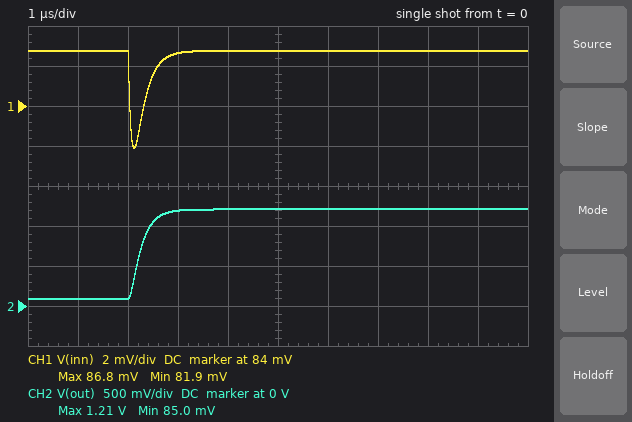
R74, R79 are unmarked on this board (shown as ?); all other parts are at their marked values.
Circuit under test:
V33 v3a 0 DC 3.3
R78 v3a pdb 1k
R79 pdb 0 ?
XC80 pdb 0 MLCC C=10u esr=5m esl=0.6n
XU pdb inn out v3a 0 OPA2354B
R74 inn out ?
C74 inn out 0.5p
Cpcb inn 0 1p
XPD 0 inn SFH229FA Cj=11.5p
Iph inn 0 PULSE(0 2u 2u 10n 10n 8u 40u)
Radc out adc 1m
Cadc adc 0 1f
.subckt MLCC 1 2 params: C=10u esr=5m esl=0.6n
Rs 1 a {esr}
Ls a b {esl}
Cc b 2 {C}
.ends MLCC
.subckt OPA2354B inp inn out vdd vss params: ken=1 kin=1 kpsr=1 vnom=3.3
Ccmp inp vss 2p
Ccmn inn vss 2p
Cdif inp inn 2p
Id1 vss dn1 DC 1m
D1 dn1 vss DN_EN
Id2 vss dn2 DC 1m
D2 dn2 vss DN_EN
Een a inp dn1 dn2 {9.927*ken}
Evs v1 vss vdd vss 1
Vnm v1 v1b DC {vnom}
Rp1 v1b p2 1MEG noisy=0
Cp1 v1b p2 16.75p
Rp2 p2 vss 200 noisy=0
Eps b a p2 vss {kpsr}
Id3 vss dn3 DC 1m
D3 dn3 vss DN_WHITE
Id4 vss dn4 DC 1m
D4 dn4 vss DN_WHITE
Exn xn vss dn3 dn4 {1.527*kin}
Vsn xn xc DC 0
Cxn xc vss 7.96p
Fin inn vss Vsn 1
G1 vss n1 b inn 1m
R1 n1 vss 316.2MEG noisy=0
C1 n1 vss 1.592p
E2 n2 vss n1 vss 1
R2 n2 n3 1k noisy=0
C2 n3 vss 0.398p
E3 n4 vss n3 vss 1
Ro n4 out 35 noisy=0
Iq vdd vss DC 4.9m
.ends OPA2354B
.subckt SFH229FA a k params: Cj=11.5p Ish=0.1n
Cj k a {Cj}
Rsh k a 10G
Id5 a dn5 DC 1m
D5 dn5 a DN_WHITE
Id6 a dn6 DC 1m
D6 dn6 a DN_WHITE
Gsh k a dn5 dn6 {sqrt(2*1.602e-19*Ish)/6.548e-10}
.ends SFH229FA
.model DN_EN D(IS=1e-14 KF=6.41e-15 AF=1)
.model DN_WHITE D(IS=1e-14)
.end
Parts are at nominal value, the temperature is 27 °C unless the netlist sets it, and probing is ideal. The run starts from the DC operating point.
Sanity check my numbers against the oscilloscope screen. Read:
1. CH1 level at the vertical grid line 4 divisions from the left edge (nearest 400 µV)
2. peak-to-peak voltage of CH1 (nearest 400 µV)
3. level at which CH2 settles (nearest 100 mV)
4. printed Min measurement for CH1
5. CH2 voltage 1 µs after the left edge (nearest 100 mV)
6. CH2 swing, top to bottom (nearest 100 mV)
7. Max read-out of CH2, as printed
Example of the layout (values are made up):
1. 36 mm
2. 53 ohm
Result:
1. 86.8 mV
2. 4.8 mV
3. 1.2 V
4. 81.9 mV
5. 100 mV
6. 1.1 V
7. 1.21 V
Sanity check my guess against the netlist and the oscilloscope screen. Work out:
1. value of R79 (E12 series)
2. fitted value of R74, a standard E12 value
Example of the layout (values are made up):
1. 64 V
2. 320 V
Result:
1. 27 Ω
2. 560 kΩ
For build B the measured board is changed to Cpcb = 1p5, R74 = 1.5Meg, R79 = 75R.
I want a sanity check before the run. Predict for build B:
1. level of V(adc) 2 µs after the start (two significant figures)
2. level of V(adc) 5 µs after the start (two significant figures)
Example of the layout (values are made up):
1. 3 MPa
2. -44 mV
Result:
1. 230 mV
2. 3.2 V
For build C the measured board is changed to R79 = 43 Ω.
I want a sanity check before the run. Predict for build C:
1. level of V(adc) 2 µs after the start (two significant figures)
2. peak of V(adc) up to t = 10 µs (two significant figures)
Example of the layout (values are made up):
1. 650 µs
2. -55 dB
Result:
1. 140 mV
2. 1.3 V
